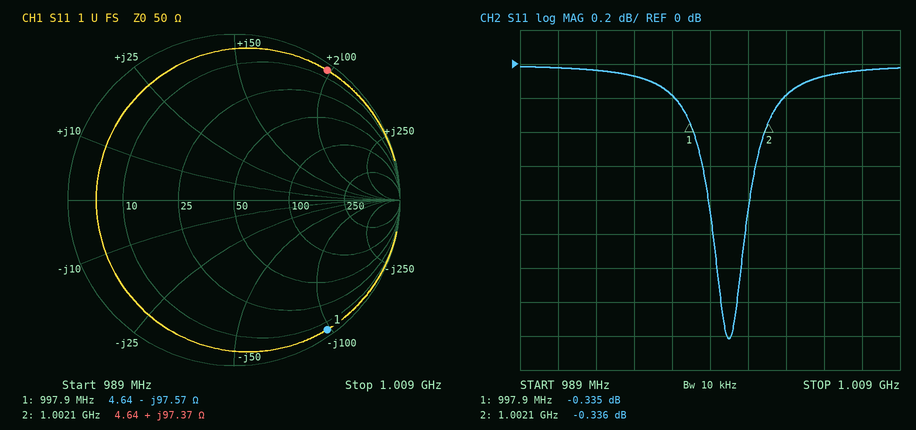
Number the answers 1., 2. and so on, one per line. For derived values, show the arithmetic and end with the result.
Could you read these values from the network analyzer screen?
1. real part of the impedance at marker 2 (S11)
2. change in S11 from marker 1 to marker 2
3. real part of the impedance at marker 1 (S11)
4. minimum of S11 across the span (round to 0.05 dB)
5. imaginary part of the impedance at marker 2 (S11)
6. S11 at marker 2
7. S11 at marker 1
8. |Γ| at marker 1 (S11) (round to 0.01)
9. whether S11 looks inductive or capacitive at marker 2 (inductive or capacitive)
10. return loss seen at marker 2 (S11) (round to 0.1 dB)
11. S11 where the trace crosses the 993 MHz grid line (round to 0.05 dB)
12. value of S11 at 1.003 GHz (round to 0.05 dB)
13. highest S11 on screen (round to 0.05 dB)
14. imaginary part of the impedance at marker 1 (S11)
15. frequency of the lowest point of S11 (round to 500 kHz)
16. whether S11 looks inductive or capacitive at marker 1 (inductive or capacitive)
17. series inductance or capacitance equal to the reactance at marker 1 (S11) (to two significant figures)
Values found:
1. 4.64 Ω
2. -0.336 − (-0.335) = -0.001 dB
3. 4.64 Ω
4. -1.60 dB
5. +97.37 Ω
6. -0.336 dB
7. -0.335 dB
8. 0.96
9. inductive
10. 0.3 dB
11. -0.05 dB
12. -0.20 dB
13. 0.00 dB
14. -97.57 Ω
15. 1.0000 GHz
16. capacitive
17. C = 1/(2π × 997.9 MHz × 97.57 Ω) ≈ 1.6 pF
